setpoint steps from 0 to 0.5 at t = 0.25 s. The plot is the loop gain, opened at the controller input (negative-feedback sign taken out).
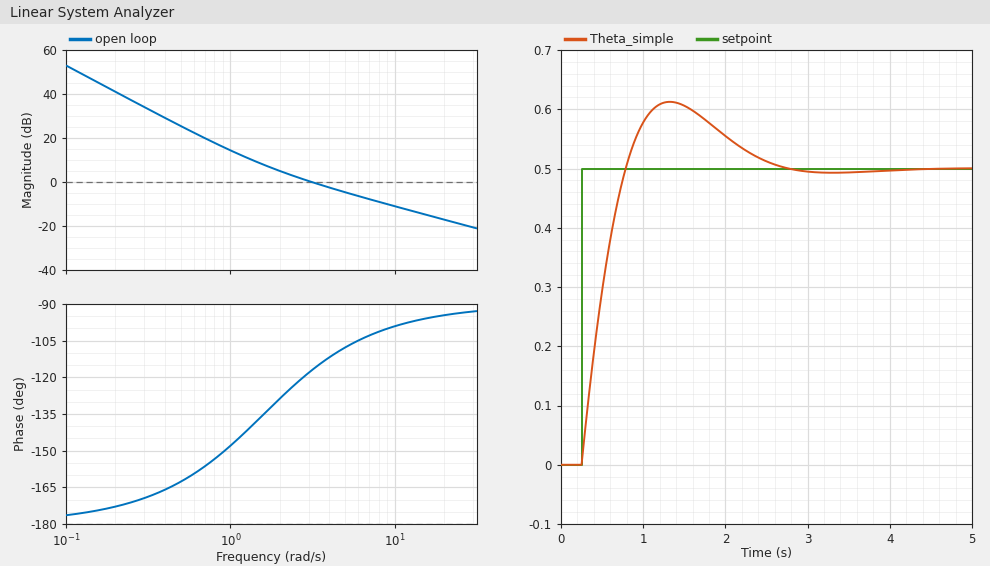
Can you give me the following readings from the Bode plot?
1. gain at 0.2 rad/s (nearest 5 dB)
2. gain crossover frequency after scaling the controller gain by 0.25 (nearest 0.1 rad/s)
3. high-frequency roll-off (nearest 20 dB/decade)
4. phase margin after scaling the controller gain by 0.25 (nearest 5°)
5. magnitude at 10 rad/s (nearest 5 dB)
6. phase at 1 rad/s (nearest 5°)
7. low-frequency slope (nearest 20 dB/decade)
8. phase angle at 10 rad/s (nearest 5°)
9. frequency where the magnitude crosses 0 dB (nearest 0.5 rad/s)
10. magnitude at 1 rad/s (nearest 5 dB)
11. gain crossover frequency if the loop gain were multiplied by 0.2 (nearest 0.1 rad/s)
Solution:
40 dB
1.2 rad/s
-20 dB/decade
35°
-10 dB
-150°
-40 dB/decade
-100°
3.0 rad/s
15 dB
1.0 rad/s
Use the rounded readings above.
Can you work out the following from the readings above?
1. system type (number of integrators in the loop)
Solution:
2
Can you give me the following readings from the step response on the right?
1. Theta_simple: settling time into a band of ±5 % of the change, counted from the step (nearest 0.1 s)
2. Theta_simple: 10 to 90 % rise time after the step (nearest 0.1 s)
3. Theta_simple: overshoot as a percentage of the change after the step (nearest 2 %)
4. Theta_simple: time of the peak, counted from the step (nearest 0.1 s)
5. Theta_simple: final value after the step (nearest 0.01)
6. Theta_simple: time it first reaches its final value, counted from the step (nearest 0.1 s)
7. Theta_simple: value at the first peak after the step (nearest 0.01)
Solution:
2.1 s
0.4 s
22 %
1.1 s
0.50
0.5 s
0.61
